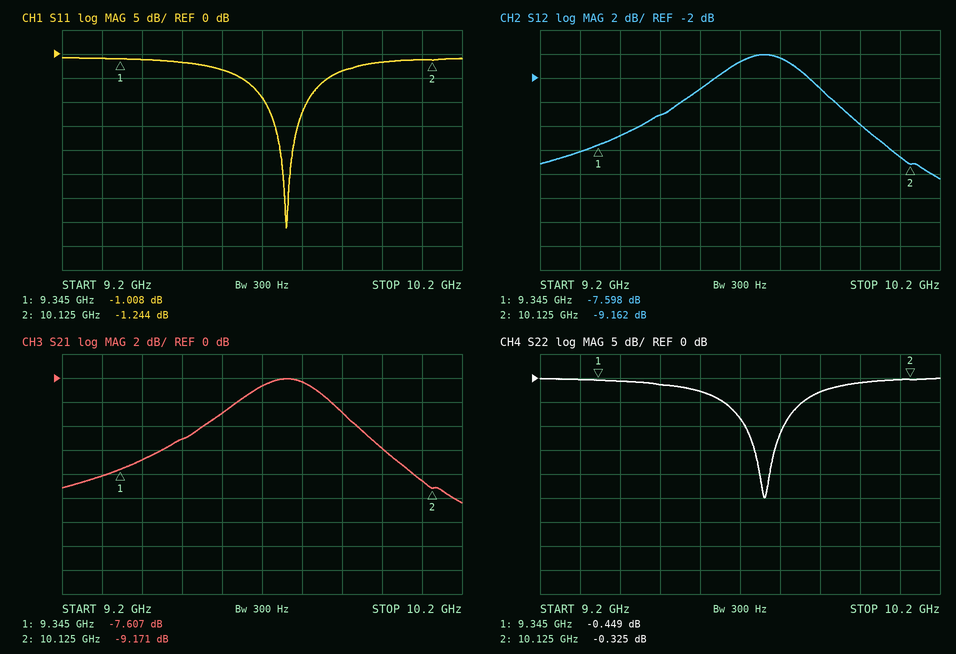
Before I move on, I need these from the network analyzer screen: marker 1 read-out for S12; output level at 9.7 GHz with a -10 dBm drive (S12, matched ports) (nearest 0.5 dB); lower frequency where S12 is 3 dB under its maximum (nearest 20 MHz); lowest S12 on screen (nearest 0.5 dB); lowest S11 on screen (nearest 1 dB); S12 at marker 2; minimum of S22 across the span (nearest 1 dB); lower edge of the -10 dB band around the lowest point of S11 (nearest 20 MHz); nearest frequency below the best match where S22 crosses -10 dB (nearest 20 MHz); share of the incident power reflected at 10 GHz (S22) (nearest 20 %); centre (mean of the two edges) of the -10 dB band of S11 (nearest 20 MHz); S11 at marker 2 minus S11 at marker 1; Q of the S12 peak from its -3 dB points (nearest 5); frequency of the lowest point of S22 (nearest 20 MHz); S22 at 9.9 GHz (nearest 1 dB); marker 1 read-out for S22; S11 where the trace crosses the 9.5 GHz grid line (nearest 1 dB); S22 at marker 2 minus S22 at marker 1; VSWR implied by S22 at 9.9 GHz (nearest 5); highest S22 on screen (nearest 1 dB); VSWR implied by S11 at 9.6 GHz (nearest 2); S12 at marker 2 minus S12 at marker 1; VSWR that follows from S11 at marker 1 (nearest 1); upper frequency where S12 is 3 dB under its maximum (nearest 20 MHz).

-7.598 dB
-10.5 dBm
9.60 GHz
-10.5 dB
-36 dB
-9.162 dB
-25 dB
9.70 GHz
9.72 GHz
80 %
9.76 GHz
-0.236 dB
30
9.76 GHz
-3 dB
-0.449 dB
-2 dB
0.124 dB
5
0 dB
6
-1.564 dB
17
9.90 GHz
